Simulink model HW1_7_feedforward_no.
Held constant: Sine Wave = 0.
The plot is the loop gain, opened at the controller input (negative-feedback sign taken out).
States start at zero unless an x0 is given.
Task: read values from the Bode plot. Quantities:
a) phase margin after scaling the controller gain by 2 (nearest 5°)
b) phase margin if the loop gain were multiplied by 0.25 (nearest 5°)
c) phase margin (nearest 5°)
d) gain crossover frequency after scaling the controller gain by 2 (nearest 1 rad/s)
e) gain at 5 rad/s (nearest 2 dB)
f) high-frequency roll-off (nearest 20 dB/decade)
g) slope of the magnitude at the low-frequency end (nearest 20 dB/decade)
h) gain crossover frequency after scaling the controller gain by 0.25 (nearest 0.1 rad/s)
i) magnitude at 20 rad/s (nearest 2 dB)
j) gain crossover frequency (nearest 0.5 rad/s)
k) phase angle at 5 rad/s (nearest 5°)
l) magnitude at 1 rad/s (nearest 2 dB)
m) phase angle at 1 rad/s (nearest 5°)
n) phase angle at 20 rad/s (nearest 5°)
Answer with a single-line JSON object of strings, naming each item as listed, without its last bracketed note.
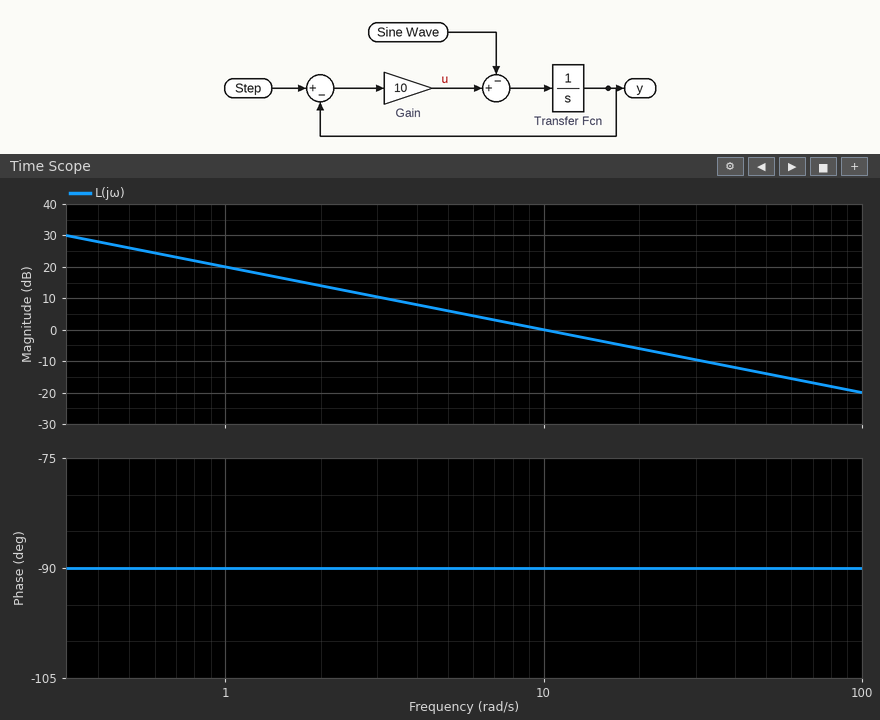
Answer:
{"phase margin after scaling the controller gain by 2": "90°", "phase margin if the loop gain were multiplied by 0.25": "90°", "phase margin": "90°", "gain crossover frequency after scaling the controller gain by 2": "20 rad/s", "gain at 5 rad/s": "6 dB", "high-frequency roll-off": "-20 dB/decade", "slope of the magnitude at the low-frequency end": "-20 dB/decade", "gain crossover frequency after scaling the controller gain by 0.25": "2.5 rad/s", "magnitude at 20 rad/s": "-6 dB", "gain crossover frequency": "10.0 rad/s", "phase angle at 5 rad/s": "-90°", "magnitude at 1 rad/s": "20 dB", "phase angle at 1 rad/s": "-90°", "phase angle at 20 rad/s": "-90°"}
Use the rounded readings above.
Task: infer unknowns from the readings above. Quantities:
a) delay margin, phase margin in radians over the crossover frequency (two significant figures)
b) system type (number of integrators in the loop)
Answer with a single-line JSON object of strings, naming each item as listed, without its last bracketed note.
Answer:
{"delay margin, phase margin in radians over the crossover frequency": "0.16 s", "system type": "1"}
